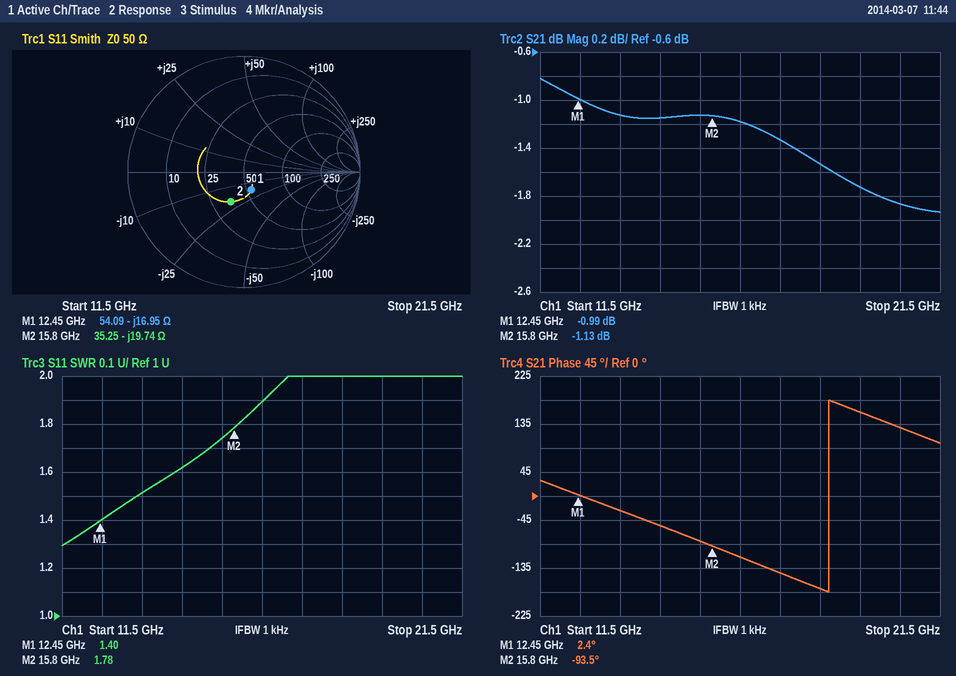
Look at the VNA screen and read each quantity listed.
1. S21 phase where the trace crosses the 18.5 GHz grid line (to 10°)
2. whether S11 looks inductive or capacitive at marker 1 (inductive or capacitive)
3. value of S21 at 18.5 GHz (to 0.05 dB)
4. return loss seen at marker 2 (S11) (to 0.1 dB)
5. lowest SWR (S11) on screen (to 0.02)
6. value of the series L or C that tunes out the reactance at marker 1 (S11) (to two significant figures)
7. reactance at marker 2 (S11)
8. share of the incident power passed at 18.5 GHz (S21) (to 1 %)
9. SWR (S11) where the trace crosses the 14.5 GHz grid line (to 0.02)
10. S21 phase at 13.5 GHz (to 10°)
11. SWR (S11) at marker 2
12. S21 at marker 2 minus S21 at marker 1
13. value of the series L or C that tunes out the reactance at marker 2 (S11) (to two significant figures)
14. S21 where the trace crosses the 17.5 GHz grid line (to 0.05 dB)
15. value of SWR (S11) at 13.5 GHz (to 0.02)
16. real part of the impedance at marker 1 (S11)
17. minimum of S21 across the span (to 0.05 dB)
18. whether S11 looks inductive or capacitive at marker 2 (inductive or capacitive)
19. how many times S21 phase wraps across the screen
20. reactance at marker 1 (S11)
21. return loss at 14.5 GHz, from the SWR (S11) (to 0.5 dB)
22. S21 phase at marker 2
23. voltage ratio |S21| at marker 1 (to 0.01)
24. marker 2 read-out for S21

-170°
capacitive
-1.55 dB
11.0 dB
1.30
220 pH
-19.74 Ω
70 %
1.62
-30°
1.78
-0.14 dB
200 pH
-1.35 dB
1.52
54.09 Ω
-1.95 dB
capacitive
1
-16.95 Ω
12.5 dB
-93.5°
0.89
-1.13 dB
